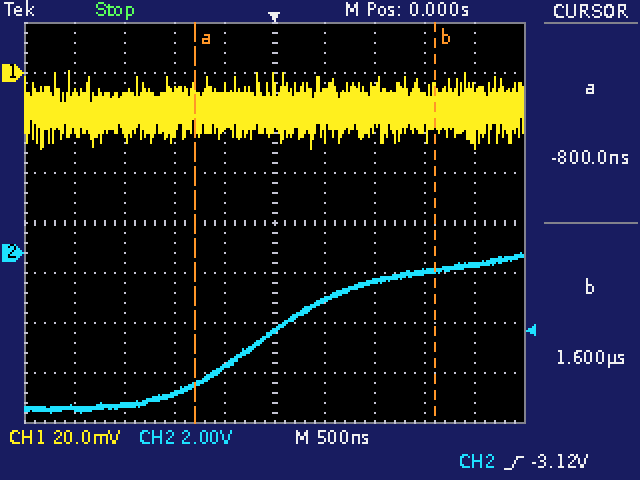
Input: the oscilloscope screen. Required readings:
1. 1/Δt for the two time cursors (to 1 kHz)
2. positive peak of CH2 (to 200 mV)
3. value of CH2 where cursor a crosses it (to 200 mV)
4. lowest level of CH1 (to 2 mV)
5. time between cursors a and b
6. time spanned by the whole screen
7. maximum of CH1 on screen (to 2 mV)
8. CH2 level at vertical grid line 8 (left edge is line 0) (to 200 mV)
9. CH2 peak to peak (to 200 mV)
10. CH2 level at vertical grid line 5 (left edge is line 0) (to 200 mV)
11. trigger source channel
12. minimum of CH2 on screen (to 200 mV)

417 kHz
0.0 V
-5.2 V
-30 mV
2.40 µs
5 µs
0 mV
-800 mV
6.4 V
-3.2 V
CH2
-6.4 V
